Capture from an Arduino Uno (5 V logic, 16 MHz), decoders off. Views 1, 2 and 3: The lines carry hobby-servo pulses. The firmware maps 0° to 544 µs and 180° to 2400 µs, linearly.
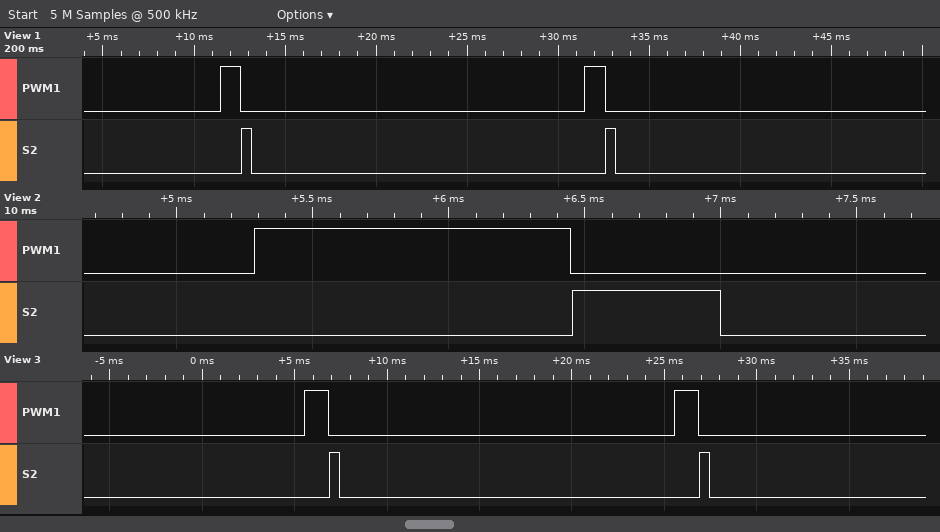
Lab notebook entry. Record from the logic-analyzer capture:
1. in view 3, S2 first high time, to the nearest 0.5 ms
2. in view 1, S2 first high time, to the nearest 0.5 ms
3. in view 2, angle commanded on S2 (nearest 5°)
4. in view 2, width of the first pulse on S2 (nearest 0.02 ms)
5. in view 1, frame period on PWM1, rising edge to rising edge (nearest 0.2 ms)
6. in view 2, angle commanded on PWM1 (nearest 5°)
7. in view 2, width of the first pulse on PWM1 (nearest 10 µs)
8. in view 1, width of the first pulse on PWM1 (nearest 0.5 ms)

0.5 ms
0.5 ms
0°
0.54 ms
20.0 ms
60°
1160 µs
1.0 ms
